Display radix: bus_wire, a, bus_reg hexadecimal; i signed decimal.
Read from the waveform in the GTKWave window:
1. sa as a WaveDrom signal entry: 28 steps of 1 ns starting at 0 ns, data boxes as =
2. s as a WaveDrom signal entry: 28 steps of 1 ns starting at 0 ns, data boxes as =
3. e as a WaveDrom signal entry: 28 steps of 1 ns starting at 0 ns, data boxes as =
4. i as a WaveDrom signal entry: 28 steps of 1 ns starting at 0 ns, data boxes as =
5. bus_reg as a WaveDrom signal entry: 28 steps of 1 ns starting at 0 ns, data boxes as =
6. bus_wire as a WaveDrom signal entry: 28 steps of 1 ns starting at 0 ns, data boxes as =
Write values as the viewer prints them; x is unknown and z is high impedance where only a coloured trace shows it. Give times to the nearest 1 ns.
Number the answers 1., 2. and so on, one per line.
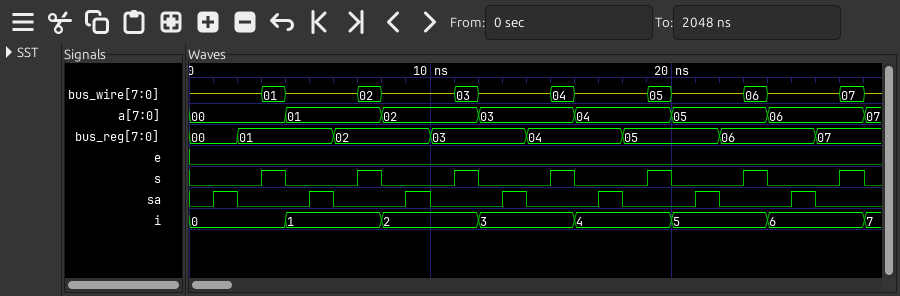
1. {name: 'sa', wave: '010..10..10..10..10..10..10.'}
2. {name: 's', wave: '0..10..10..10..10..10..10..1'}
3. {name: 'e', wave: '0...........................'}
4. {name: 'i', wave: '=...=...=...=...=...=...=...', data: '0 1 2 3 4 5 6'}
5. {name: 'bus_reg', wave: '=.=...=...=...=...=...=...=.', data: '00 01 02 03 04 05 06 07'}
6. {name: 'bus_wire', wave: 'z..=z..=z..=z..=z..=z..=z..=', data: '01 02 03 04 05 06 07'}
